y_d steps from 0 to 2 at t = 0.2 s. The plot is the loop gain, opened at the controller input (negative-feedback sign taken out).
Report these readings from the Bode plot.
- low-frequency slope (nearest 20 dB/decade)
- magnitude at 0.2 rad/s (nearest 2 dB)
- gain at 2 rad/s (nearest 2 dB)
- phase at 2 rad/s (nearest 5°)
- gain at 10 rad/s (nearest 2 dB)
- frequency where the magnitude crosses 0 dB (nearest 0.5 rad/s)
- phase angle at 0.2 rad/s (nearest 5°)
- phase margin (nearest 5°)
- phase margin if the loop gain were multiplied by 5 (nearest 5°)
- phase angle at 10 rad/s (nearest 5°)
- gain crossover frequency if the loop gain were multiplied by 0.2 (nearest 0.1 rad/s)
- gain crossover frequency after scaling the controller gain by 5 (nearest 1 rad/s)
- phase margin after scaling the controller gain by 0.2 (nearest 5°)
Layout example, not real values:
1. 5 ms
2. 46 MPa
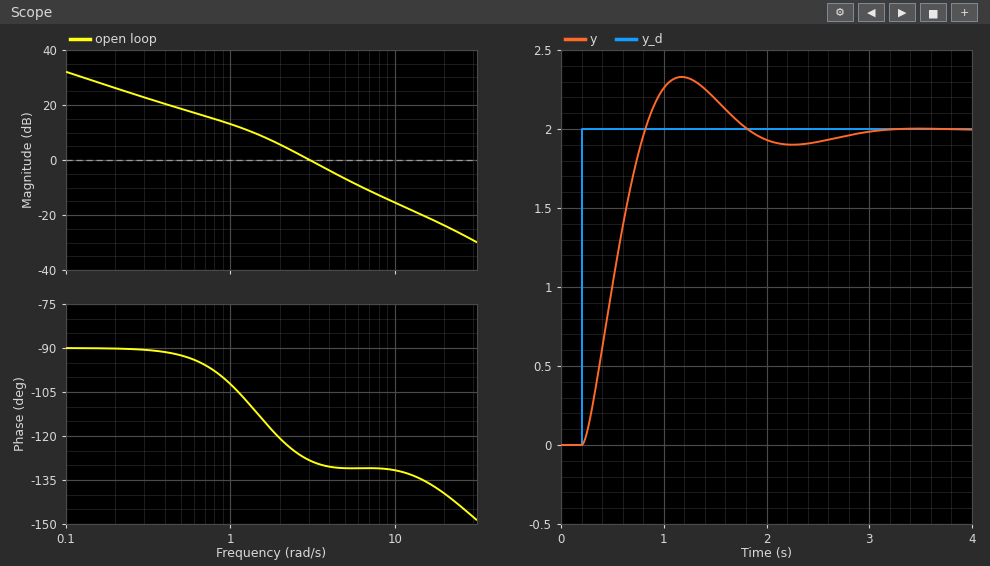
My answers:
1. -20 dB/decade
2. 26 dB
3. 6 dB
4. -120°
5. -16 dB
6. 3.0 rad/s
7. -90°
8. 50°
9. 50°
10. -130°
11. 0.9 rad/s
12. 9 rad/s
13. 80°
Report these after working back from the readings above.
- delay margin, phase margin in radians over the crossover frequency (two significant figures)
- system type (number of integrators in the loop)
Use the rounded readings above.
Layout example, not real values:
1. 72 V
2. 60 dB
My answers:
1. 0.29 s
2. 1
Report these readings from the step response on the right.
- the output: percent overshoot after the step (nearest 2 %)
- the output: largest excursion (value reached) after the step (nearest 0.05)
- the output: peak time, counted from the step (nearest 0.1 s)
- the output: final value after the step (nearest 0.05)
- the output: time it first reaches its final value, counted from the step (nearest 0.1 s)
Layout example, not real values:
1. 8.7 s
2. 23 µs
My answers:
1. 16 %
2. 2.35
3. 1.0 s
4. 2.00
5. 0.6 s
